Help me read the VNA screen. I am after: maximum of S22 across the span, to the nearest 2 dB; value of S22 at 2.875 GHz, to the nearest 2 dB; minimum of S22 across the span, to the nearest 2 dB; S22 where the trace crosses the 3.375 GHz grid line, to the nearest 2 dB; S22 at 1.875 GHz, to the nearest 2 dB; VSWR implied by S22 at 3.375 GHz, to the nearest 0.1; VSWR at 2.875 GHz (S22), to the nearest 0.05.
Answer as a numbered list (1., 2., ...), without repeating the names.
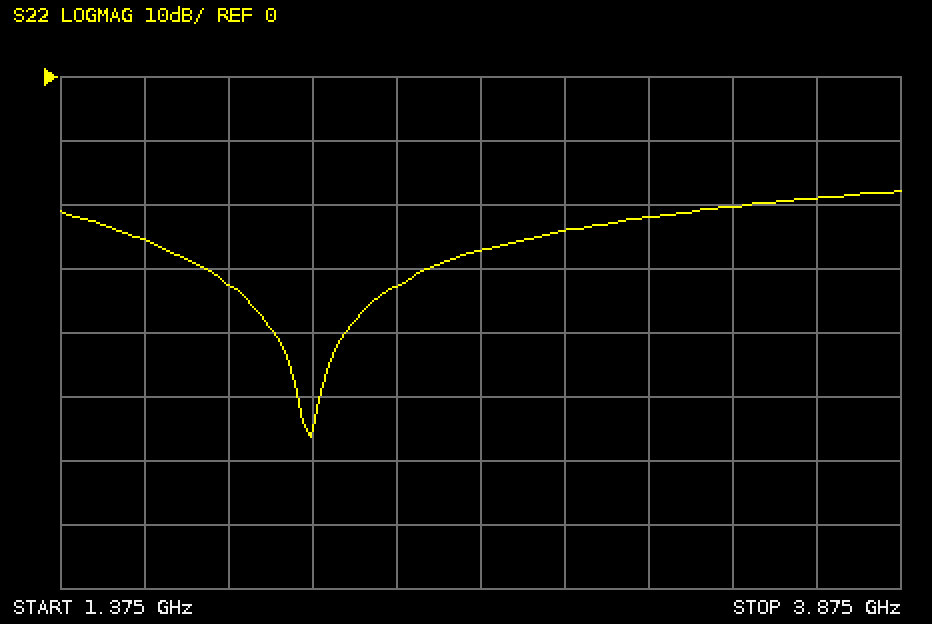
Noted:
1. -18 dB
2. -24 dB
3. -56 dB
4. -20 dB
5. -32 dB
6. 1.2
7. 1.15
